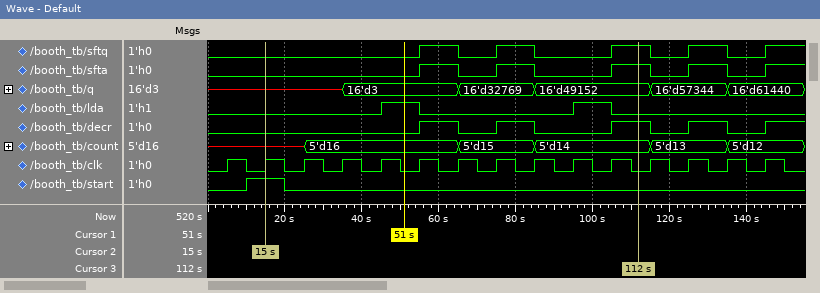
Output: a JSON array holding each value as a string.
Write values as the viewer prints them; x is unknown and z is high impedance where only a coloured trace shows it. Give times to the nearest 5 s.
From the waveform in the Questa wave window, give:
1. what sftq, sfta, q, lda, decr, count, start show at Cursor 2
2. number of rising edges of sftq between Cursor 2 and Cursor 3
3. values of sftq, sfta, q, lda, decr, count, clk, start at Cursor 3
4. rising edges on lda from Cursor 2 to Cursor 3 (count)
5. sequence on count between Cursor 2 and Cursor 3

["sftq=0, sfta=0, q=x, lda=0, decr=0, count=x, start=1", "3", "sftq=1, sfta=1, q=16'd49152, lda=0, decr=1, count=5'd14, clk=0, start=0", "2", "x, 5'd16, 5'd15, 5'd14"]
